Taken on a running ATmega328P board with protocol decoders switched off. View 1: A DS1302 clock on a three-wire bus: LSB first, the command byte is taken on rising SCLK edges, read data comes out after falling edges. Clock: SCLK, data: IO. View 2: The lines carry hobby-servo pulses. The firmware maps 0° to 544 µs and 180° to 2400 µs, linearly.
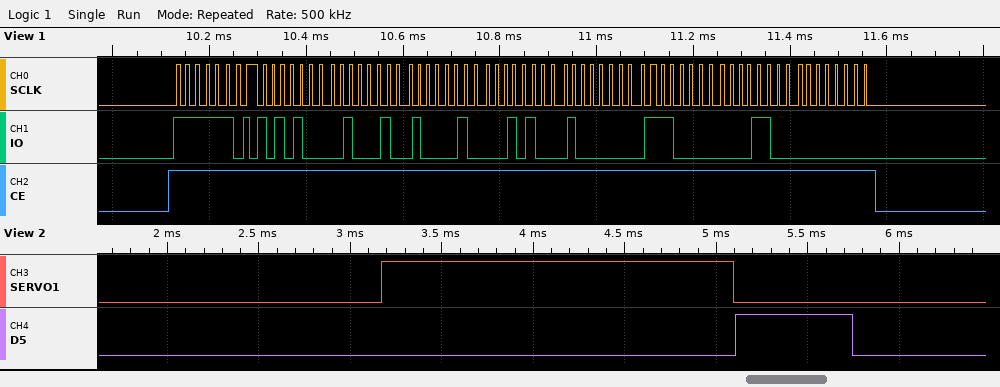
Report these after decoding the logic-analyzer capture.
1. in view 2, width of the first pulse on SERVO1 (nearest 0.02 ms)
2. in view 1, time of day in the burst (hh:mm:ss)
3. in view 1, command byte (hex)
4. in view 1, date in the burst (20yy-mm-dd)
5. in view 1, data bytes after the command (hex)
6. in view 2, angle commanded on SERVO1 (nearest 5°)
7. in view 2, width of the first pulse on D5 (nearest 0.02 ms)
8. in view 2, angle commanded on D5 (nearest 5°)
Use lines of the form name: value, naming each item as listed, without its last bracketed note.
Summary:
in view 2, width of the first pulse on SERVO1: 1.92 ms
in view 1, time of day in the burst: 21:22:15
in view 1, command byte: 0xBF
in view 1, date in the burst: 2018-01-14
in view 1, data bytes after the command: 15 22 21 14 01 07 18 00
in view 2, angle commanded on SERVO1: 135°
in view 2, width of the first pulse on D5: 0.64 ms
in view 2, angle commanded on D5: 10°
